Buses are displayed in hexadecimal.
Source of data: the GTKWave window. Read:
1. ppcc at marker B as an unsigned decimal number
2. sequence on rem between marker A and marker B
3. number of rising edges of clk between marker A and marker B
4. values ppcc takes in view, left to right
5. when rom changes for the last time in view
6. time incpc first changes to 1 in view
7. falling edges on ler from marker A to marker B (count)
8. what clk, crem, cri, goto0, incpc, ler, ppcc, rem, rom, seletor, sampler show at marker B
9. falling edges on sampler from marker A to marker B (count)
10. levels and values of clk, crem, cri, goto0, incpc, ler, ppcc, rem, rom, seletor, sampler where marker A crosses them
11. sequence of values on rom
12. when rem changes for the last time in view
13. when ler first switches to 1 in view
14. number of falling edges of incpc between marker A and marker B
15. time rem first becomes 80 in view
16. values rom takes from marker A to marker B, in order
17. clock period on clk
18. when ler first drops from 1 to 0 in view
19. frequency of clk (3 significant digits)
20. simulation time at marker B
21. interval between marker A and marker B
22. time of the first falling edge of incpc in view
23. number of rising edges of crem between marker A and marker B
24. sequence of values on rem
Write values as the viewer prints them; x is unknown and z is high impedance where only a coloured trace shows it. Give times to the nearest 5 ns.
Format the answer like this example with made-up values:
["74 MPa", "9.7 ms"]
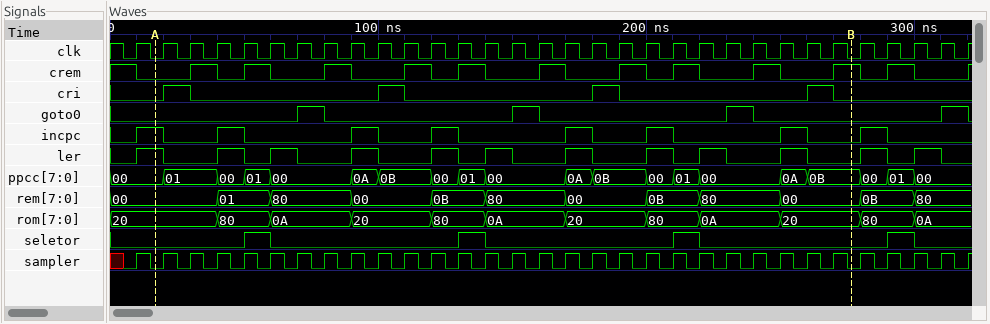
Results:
["11", "00, 01, 80, 00, 0B, 80, 00, 0B, 80, 00", "26", "00, 01, 00, 01, 00, 0A, 0B, 00, 01, 00, 0A, 0B, 00, 01, 00, 0A, 0B, 00, 01, 00", "300 ns", "10 ns", "10", "clk=0, crem=1, cri=0, goto0=0, incpc=0, ler=0, ppcc=0B, rem=00, rom=20, seletor=0, sampler=0", "26", "clk=0, crem=0, cri=0, goto0=0, incpc=1, ler=1, ppcc=00, rem=00, rom=20, seletor=0, sampler=0", "20, 80, 0A, 20, 80, 0A, 20, 80, 0A, 20, 80, 0A", "300 ns", "10 ns", "7", "60 ns", "20, 80, 0A, 20, 80, 0A, 20, 80, 0A, 20", "10 ns", "20 ns", "100 MHz", "275 ns", "260 ns", "20 ns", "10", "00, 01, 80, 00, 0B, 80, 00, 0B, 80, 00, 0B, 80"]
